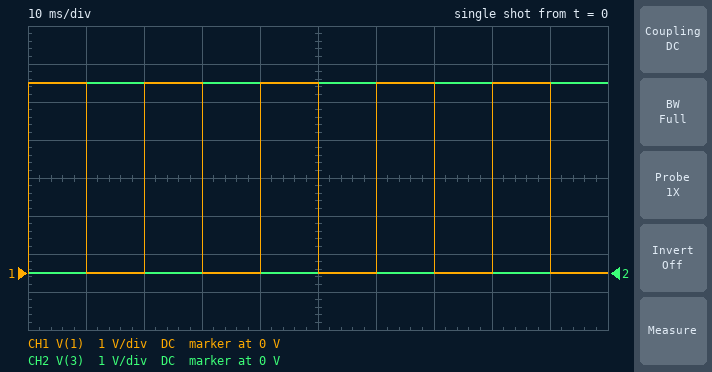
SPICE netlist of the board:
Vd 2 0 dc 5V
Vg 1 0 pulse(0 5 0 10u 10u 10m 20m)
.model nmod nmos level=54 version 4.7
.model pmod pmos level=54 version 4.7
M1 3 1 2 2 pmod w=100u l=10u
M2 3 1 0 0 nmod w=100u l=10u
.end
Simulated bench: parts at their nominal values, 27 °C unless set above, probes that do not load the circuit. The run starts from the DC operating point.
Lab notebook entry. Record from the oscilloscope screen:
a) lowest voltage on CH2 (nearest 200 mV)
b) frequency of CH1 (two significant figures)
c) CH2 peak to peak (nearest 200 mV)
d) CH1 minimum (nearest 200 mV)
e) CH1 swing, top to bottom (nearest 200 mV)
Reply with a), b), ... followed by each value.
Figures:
a) 0 V
b) 50 Hz
c) 5.0 V
d) 0 V
e) 5.0 V
